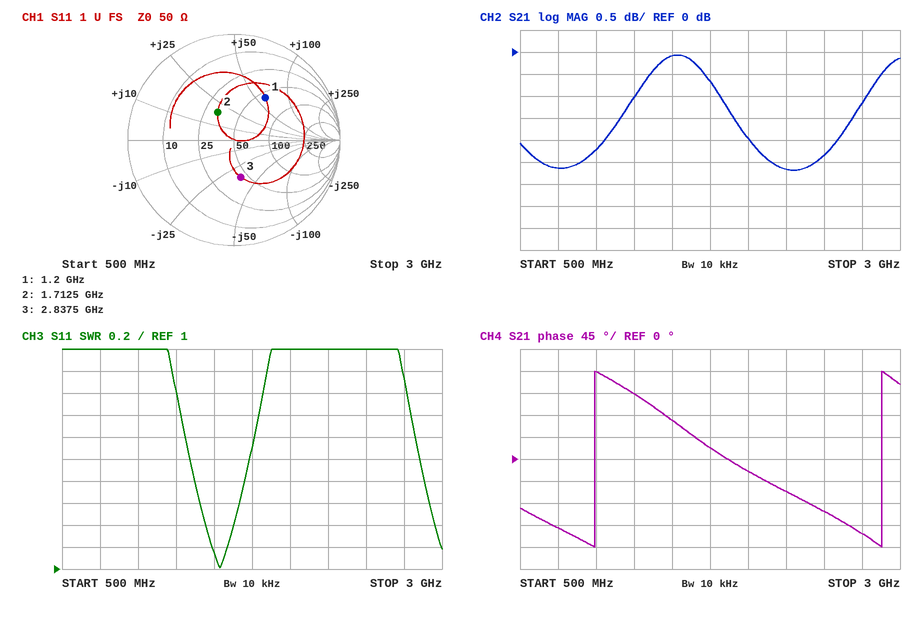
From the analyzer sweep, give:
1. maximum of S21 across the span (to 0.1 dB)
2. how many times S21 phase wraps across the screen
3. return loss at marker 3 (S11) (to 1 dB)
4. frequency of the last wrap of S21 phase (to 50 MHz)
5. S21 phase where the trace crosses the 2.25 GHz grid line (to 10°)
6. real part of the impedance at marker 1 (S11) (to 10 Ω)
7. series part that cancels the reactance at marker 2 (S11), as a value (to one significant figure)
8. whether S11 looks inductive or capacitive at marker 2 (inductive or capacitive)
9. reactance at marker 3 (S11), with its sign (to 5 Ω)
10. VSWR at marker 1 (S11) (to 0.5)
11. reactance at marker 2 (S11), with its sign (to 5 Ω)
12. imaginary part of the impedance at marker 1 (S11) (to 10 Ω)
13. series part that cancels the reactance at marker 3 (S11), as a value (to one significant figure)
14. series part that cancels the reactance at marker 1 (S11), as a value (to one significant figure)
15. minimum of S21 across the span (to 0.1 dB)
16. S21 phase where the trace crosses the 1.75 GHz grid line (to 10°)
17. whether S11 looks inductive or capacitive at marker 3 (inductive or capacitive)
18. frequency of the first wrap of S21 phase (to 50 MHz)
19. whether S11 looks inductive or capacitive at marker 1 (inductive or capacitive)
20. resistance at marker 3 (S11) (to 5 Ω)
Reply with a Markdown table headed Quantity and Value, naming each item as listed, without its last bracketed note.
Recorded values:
| Quantity | Value |
|---|---|
| maximum of S21 across the span | -0.1 dB |
| how many times S21 phase wraps across the screen | 2 |
| return loss at marker 3 (S11) | 9 dB |
| frequency of the last wrap of S21 phase | 2.90 GHz |
| S21 phase where the trace crosses the 2.25 GHz grid line | -70° |
| real part of the impedance at marker 1 (S11) | 60 Ω |
| series part that cancels the reactance at marker 2 (S11), as a value | 5 pF |
| whether S11 looks inductive or capacitive at marker 2 | inductive |
| reactance at marker 3 (S11), with its sign | -35 Ω |
| VSWR at marker 1 (S11) | 3.0 |
| reactance at marker 2 (S11), with its sign | +20 Ω |
| imaginary part of the impedance at marker 1 (S11) | +60 Ω |
| series part that cancels the reactance at marker 3 (S11), as a value | 2 nH |
| series part that cancels the reactance at marker 1 (S11), as a value | 2 pF |
| minimum of S21 across the span | -2.7 dB |
| S21 phase where the trace crosses the 1.75 GHz grid line | 20° |
| whether S11 looks inductive or capacitive at marker 3 | capacitive |
| frequency of the first wrap of S21 phase | 1.00 GHz |
| whether S11 looks inductive or capacitive at marker 1 | inductive |
| resistance at marker 3 (S11) | 45 Ω |
